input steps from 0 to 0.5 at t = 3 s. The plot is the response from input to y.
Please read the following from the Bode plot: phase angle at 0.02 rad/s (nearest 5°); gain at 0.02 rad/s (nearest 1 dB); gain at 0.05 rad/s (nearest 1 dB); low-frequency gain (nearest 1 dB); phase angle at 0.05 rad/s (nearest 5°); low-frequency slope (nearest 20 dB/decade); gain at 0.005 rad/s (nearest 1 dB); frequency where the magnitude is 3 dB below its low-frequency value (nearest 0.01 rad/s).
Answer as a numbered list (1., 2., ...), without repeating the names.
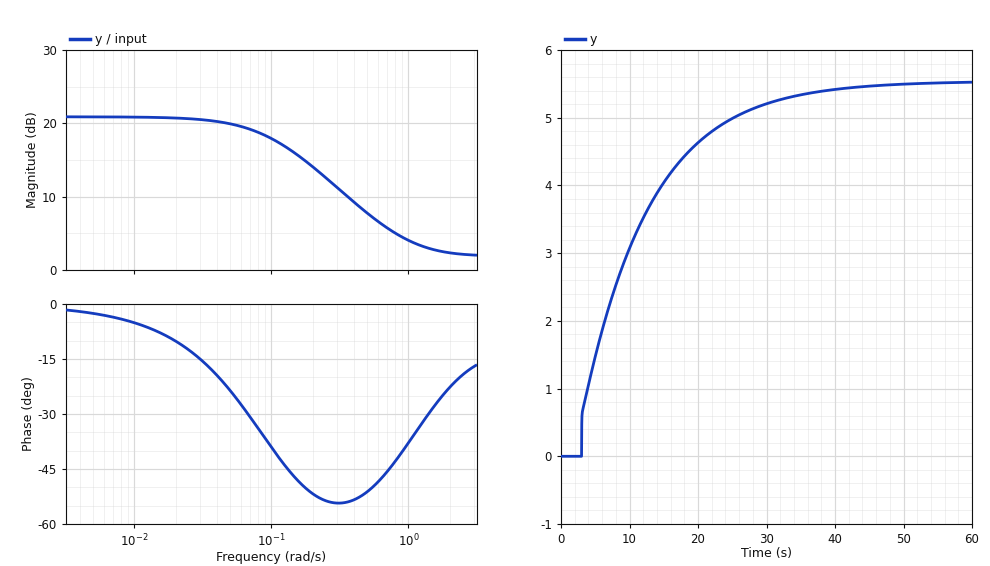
1. -10°
2. 21 dB
3. 20 dB
4. 21 dB
5. -25°
6. 0 dB/decade
7. 21 dB
8. 0.10 rad/s
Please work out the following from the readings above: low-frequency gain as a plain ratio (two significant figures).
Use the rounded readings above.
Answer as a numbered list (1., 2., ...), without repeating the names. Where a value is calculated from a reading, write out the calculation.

1. 10^(21 / 20) = 11
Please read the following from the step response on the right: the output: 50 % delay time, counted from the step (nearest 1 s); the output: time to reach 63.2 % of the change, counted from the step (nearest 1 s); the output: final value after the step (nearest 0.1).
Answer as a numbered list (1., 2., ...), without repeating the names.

1. 6 s
2. 9 s
3. 5.5
